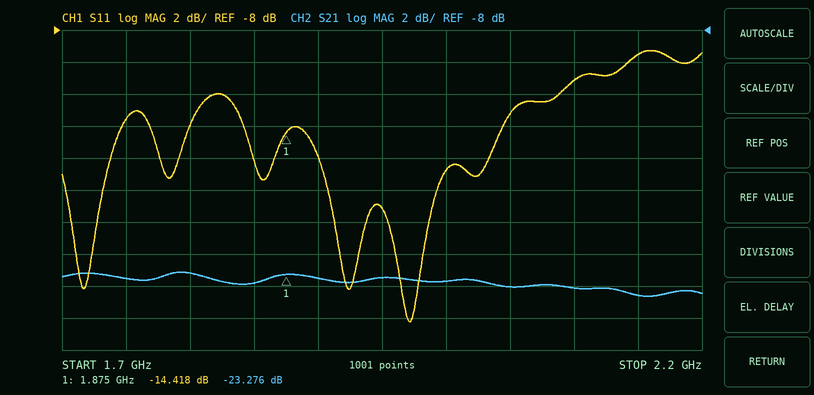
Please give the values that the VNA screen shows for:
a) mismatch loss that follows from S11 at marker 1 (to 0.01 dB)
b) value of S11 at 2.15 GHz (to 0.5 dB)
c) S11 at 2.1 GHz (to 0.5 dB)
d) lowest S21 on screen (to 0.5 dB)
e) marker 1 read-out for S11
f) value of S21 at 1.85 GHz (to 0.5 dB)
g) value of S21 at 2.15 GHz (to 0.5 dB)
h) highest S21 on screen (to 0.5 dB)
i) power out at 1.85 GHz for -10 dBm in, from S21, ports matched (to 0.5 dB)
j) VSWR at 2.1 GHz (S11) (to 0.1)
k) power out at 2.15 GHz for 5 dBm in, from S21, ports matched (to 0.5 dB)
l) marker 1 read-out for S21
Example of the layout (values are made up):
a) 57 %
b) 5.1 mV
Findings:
a) 0.16 dB
b) -9.5 dB
c) -11.0 dB
d) -24.5 dB
e) -14.418 dB
f) -24.0 dB
g) -24.5 dB
h) -23.0 dB
i) -34.0 dBm
j) 1.8
k) -19.5 dBm
l) -23.276 dB
